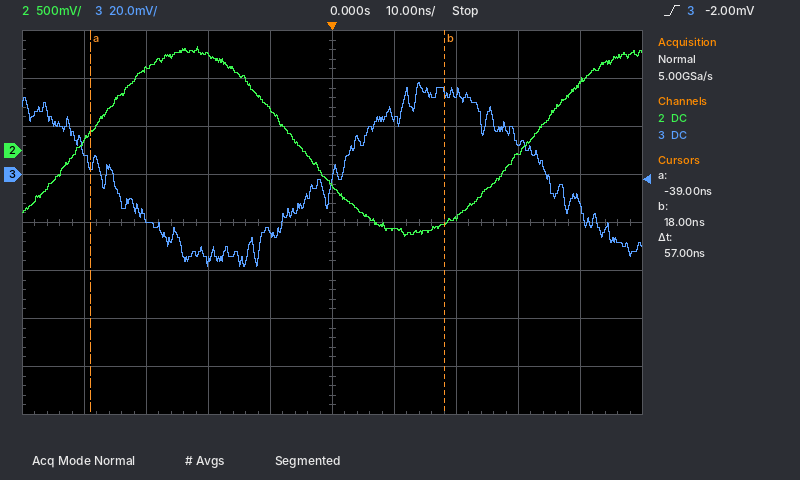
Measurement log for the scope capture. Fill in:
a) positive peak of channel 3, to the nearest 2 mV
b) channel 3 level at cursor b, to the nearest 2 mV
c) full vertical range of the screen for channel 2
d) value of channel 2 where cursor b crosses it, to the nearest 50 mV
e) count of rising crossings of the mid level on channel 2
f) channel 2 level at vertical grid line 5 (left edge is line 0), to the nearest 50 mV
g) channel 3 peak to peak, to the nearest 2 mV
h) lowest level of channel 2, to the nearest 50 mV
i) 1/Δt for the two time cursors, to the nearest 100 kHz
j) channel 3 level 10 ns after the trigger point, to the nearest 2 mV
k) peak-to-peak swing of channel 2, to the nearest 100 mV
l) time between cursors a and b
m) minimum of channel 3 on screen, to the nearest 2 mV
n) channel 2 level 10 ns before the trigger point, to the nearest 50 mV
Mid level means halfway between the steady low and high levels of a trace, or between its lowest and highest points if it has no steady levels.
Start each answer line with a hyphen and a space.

- 38 mV
- 34 mV
- 4 V
- -750 mV
- 2
- -350 mV
- 76 mV
- -900 mV
- 17.5 MHz
- 24 mV
- 2.00 V
- 57 ns
- -38 mV
- 450 mV
